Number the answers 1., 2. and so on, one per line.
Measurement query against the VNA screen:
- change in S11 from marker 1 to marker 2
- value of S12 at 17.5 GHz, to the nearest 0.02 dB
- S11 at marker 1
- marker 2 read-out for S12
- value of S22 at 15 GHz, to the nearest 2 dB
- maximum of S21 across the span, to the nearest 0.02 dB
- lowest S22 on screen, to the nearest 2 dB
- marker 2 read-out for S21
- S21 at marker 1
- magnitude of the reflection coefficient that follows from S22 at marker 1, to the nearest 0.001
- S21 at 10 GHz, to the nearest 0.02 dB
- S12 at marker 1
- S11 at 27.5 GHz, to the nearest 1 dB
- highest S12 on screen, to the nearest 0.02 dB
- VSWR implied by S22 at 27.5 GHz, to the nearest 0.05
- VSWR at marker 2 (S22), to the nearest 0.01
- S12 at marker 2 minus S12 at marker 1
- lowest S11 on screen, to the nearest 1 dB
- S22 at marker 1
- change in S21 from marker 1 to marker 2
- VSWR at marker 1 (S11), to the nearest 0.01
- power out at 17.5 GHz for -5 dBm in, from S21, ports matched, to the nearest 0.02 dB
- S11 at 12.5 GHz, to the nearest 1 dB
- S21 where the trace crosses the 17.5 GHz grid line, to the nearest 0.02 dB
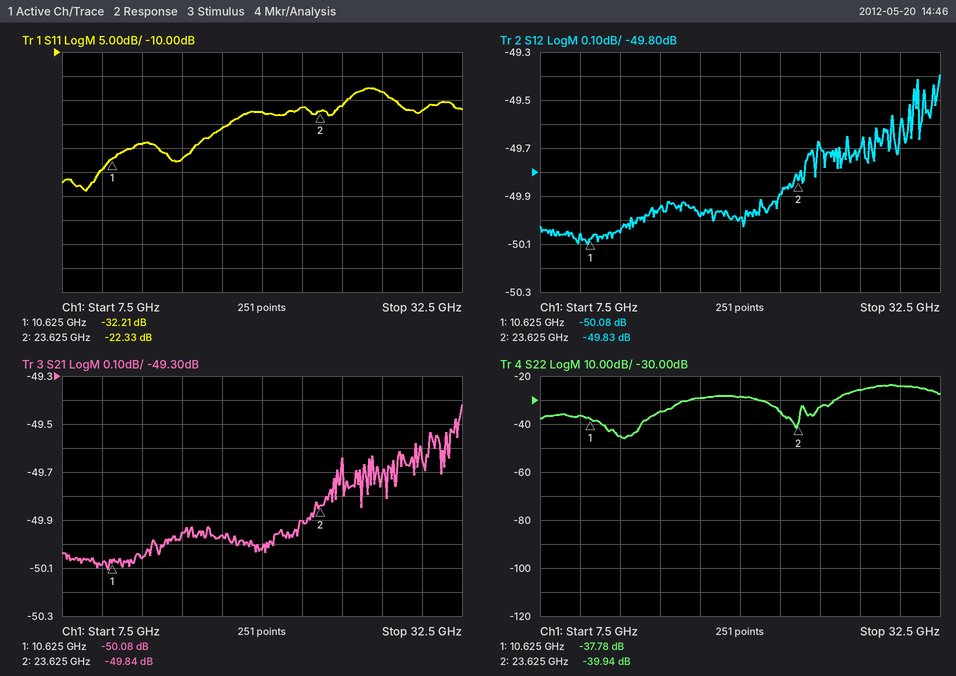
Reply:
1. 9.88 dB
2. -49.98 dB
3. -32.21 dB
4. -49.83 dB
5. -34 dB
6. -49.42 dB
7. -46 dB
8. -49.84 dB
9. -50.08 dB
10. 0.013
11. -50.08 dB
12. -50.08 dB
13. -18 dB
14. -49.40 dB
15. 1.10
16. 1.02
17. 0.25 dB
18. -39 dB
19. -37.78 dB
20. 0.24 dB
21. 1.05
22. -54.96 dBm
23. -29 dB
24. -49.96 dB
